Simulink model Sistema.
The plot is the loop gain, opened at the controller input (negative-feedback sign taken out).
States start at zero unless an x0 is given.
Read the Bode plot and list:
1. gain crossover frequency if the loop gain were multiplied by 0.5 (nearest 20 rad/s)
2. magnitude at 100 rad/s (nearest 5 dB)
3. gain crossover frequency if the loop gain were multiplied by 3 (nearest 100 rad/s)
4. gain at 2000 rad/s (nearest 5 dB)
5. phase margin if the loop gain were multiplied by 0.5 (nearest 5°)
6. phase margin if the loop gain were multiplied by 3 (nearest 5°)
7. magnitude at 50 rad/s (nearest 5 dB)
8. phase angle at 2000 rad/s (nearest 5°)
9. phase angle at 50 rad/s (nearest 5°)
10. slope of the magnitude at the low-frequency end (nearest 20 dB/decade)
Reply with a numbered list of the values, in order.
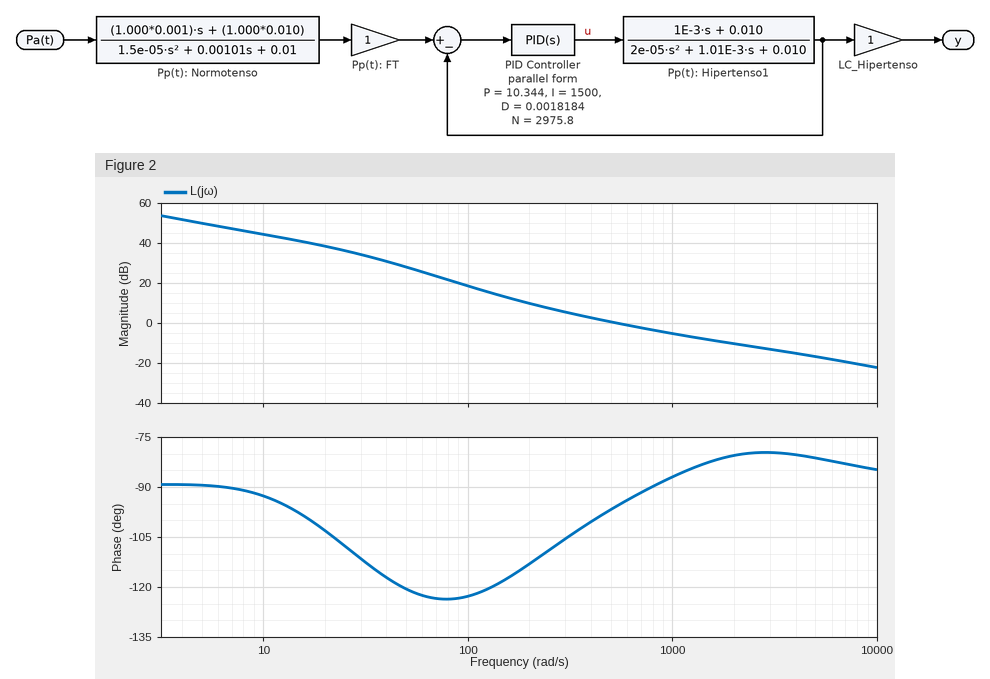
1. 280 rad/s
2. 20 dB
3. 1800 rad/s
4. -10 dB
5. 75°
6. 100°
7. 30 dB
8. -80°
9. -120°
10. -20 dB/decade
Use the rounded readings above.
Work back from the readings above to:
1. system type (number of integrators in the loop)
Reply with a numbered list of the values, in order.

1. 1
